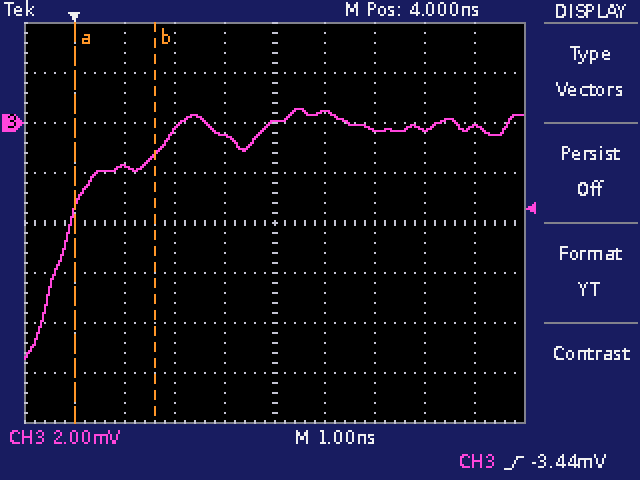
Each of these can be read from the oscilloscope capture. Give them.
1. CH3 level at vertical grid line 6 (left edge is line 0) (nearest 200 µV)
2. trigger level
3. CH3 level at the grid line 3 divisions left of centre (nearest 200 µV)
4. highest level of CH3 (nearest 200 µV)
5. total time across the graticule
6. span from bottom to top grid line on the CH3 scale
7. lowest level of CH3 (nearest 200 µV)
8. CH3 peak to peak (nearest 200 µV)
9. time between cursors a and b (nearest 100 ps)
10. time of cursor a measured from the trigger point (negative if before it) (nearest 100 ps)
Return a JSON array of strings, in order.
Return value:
["400 µV", "-3.44 mV", "-1.8 mV", "600 µV", "10 ns", "16 mV", "-9.4 mV", "10.0 mV", "1.6 ns", "0.0 ns"]
